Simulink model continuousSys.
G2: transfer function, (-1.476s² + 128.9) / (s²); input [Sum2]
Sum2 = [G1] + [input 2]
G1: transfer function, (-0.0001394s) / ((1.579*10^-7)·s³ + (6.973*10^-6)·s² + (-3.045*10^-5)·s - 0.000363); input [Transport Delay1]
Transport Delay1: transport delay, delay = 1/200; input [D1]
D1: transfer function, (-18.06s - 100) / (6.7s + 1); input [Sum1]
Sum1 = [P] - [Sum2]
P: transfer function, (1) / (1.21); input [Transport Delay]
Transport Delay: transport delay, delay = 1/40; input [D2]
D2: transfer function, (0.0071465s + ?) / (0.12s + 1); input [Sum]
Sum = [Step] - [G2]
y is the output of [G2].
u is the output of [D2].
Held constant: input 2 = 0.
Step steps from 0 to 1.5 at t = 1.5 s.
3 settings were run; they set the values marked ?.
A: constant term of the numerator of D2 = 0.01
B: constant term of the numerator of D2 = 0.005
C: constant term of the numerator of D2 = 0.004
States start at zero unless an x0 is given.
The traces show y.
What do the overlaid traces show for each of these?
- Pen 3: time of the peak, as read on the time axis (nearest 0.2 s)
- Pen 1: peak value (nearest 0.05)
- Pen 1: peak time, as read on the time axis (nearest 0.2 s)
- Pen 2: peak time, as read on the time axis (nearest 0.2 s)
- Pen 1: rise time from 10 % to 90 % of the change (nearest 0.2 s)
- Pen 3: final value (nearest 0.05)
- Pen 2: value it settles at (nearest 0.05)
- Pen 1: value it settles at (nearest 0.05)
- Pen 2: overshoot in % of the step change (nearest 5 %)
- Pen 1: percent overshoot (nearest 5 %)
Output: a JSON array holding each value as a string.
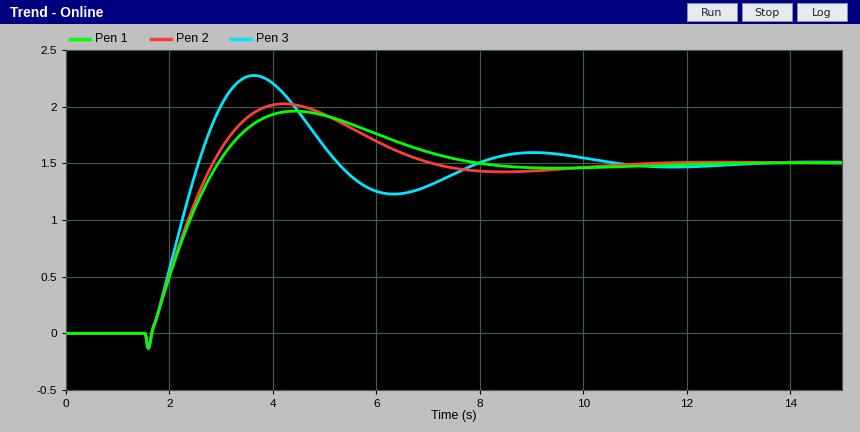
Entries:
["3.6 s", "1.95", "4.4 s", "4.2 s", "1.0 s", "1.50", "1.50", "1.50", "35 %", "30 %"]
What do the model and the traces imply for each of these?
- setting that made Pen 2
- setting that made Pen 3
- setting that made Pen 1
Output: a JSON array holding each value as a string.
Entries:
["B", "A", "C"]
